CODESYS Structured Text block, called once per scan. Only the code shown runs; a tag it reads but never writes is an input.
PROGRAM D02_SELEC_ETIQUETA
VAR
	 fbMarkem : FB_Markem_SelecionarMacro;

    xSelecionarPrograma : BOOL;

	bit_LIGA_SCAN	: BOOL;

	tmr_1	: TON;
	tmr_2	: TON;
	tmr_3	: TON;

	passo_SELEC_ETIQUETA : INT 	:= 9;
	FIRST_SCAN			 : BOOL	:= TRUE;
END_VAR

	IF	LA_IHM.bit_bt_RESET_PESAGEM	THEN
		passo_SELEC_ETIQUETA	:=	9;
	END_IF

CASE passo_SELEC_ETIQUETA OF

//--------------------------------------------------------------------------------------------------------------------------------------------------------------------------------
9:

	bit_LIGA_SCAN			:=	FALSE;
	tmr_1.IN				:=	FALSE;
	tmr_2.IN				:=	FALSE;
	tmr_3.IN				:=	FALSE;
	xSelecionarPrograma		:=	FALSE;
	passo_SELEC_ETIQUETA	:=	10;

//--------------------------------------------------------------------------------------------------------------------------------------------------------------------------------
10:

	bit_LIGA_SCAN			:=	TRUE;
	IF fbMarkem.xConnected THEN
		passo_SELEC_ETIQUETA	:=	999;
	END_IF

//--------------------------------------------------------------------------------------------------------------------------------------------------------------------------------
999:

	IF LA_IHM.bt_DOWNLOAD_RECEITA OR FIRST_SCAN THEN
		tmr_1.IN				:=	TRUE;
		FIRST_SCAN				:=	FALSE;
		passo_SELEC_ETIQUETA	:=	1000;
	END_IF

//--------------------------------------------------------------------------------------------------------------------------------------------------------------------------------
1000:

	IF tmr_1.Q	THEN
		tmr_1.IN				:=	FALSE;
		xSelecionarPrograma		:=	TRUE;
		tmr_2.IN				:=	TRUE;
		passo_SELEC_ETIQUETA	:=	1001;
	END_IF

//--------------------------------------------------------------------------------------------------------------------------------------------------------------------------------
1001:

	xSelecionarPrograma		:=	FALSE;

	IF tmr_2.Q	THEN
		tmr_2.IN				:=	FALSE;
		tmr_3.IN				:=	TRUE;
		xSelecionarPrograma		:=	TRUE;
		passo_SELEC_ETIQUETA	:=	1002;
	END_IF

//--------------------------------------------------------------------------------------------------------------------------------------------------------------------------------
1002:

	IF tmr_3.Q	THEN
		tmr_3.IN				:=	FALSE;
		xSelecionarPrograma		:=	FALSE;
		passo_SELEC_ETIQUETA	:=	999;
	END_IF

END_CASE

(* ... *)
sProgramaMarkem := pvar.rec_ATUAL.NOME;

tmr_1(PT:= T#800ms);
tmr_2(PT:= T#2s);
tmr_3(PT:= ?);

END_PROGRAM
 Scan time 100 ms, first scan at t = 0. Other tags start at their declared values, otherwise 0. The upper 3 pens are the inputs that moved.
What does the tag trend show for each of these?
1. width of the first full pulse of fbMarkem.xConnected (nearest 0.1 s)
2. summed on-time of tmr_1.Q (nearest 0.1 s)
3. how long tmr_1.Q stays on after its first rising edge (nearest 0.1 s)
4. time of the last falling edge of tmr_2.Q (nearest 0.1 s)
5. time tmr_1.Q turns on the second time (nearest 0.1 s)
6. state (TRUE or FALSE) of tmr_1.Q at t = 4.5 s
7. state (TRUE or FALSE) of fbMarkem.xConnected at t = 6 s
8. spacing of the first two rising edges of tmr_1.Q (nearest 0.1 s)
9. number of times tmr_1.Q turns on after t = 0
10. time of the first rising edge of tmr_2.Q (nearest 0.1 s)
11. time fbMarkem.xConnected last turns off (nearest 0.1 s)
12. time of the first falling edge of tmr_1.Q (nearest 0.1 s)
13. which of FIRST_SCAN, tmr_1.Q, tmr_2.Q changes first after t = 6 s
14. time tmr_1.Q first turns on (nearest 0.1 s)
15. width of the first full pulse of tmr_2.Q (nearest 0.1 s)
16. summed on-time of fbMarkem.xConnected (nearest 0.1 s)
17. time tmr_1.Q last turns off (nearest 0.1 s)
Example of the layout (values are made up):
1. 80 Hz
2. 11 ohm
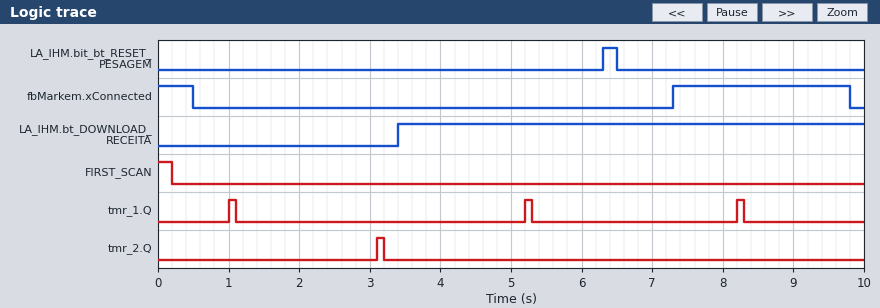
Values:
1. 2.5 s
2. 0.3 s
3. 0.1 s
4. 3.2 s
5. 5.2 s
6. FALSE
7. FALSE
8. 4.2 s
9. 3
10. 3.1 s
11. 9.8 s
12. 1.1 s
13. tmr_1.Q
14. 1.0 s
15. 0.1 s
16. 3.0 s
17. 8.3 s
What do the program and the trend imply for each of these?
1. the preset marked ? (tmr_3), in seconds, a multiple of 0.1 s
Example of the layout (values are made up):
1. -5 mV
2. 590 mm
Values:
1. 1.0 s
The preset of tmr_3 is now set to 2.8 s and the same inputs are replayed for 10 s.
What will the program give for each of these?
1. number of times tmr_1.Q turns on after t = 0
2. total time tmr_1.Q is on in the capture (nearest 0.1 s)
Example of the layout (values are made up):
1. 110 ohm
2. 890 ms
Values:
1. 2
2. 0.2 s
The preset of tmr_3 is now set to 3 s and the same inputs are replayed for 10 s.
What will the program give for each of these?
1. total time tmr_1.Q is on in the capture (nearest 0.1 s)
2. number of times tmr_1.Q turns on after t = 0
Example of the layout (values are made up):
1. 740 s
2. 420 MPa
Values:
1. 0.2 s
2. 2
